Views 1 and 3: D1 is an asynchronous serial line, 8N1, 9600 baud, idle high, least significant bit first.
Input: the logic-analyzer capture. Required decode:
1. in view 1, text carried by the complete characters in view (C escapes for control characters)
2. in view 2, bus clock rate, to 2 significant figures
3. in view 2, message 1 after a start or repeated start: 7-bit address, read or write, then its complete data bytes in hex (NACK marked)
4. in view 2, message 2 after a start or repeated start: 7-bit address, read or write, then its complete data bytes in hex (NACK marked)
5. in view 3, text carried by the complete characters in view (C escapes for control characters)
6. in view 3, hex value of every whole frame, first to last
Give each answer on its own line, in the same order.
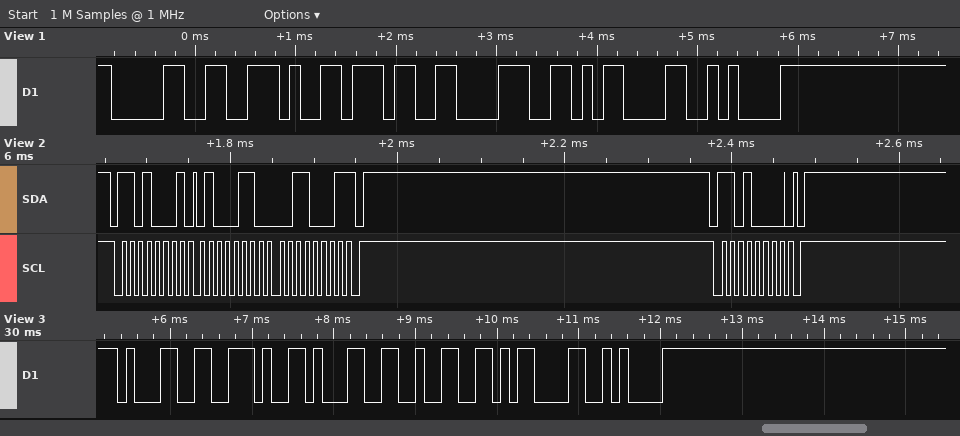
"0.78\r\n"
100 kHz
0x68 read: 46 31 NACK
0x68 write
"1.12\r\n"
0x31 0x2E 0x31 0x32 0x0D 0x0A
